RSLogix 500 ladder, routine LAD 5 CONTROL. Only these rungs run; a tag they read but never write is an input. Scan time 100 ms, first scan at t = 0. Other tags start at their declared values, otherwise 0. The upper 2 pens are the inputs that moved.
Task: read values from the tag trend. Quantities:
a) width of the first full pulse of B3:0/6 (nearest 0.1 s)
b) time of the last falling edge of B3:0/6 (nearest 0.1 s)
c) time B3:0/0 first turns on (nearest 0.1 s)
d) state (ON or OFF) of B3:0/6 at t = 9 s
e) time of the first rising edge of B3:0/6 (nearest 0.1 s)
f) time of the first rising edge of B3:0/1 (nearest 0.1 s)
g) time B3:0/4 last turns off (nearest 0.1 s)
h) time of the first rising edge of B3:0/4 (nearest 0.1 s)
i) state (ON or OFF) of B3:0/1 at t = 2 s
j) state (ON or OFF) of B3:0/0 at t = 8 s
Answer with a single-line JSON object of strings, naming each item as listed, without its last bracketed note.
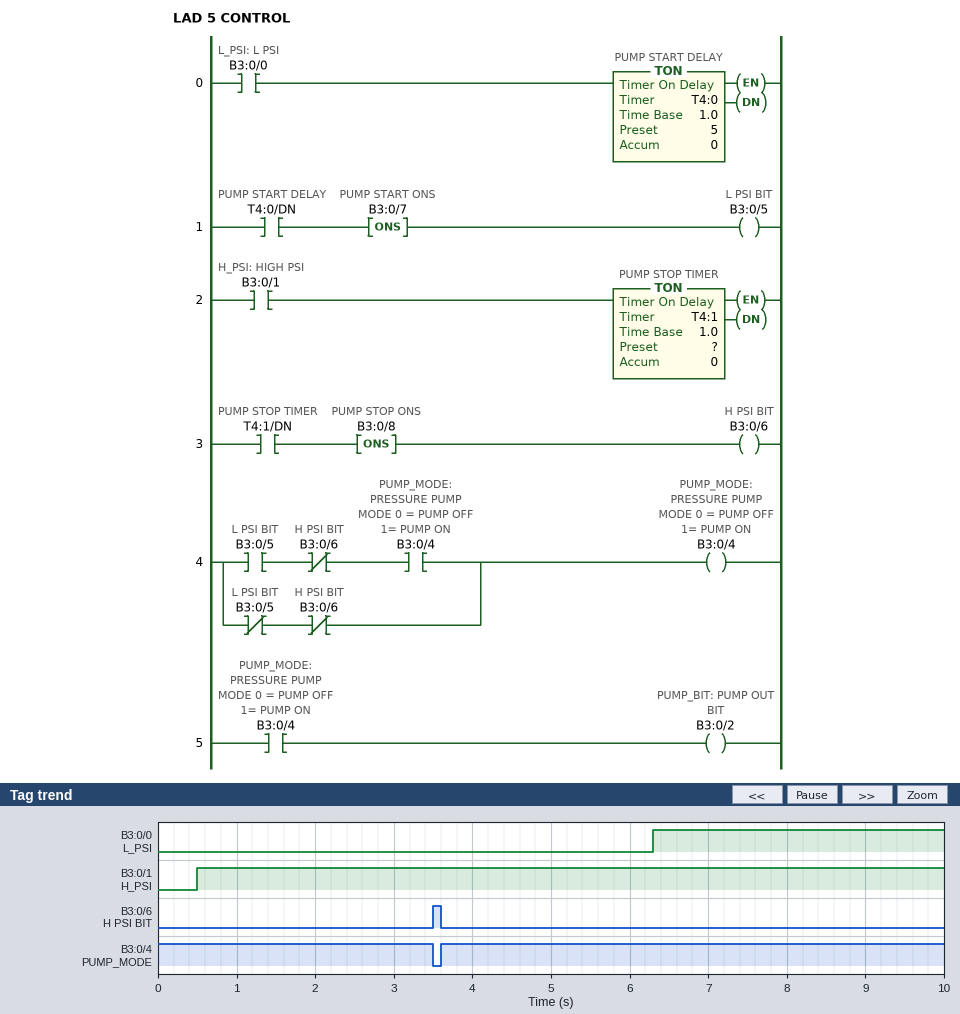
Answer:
{"width of the first full pulse of B3:0/6": "0.1 s", "time of the last falling edge of B3:0/6": "3.6 s", "time B3:0/0 first turns on": "6.3 s", "state (ON or OFF) of B3:0/6 at t = 9 s": "OFF", "time of the first rising edge of B3:0/6": "3.5 s", "time of the first rising edge of B3:0/1": "0.5 s", "time B3:0/4 last turns off": "3.5 s", "time of the first rising edge of B3:0/4": "3.6 s", "state (ON or OFF) of B3:0/1 at t = 2 s": "ON", "state (ON or OFF) of B3:0/0 at t = 8 s": "ON"}
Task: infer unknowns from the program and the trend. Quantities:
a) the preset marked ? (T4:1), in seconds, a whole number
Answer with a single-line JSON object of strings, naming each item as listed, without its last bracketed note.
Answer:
{"the preset marked ? (T4:1), in seconds, a whole number": "3 s"}
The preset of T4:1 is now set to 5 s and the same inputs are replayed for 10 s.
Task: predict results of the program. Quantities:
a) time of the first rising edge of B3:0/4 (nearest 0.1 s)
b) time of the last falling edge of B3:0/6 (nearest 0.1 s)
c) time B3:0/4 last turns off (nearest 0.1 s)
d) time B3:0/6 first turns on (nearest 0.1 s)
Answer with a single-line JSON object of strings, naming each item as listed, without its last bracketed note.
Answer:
{"time of the first rising edge of B3:0/4": "5.6 s", "time of the last falling edge of B3:0/6": "5.6 s", "time B3:0/4 last turns off": "5.5 s", "time B3:0/6 first turns on": "5.5 s"}
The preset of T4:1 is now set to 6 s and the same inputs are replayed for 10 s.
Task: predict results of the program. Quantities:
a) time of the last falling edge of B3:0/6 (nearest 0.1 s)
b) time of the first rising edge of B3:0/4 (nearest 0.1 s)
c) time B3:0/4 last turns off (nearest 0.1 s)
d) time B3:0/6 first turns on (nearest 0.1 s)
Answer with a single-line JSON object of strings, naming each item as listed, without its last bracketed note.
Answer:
{"time of the last falling edge of B3:0/6": "6.6 s", "time of the first rising edge of B3:0/4": "6.6 s", "time B3:0/4 last turns off": "6.5 s", "time B3:0/6 first turns on": "6.5 s"}
